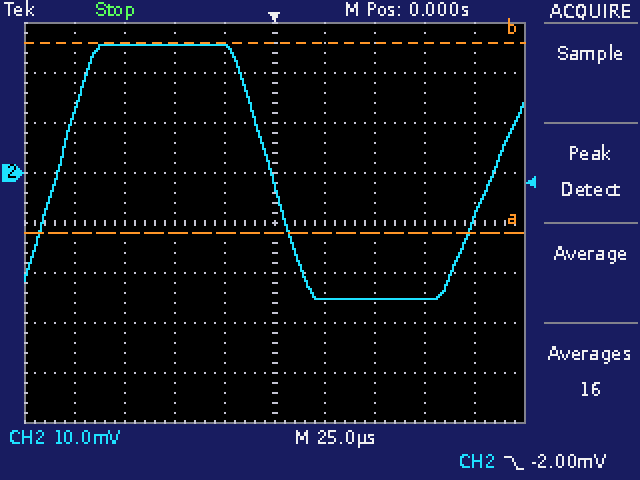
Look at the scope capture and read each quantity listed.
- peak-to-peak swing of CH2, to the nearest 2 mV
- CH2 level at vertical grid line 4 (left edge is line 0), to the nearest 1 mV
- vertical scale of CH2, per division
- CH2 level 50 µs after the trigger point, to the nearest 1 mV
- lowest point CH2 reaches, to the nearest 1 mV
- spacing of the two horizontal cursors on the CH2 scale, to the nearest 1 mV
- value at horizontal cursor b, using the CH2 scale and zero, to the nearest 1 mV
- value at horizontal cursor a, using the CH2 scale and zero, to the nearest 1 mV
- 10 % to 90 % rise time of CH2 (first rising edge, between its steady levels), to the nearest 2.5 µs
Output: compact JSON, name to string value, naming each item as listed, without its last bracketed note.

{"peak-to-peak swing of CH2, to the nearest 2 mV": "50 mV", "CH2 level at vertical grid line 4 (left edge is line 0), to the nearest 1 mV": "25 mV", "vertical scale of CH2, per division": "10 mV", "CH2 level 50 µs after the trigger point, to the nearest 1 mV": "-25 mV", "lowest point CH2 reaches, to the nearest 1 mV": "-25 mV", "spacing of the two horizontal cursors on the CH2 scale, to the nearest 1 mV": "38 mV", "value at horizontal cursor b, using the CH2 scale and zero, to the nearest 1 mV": "26 mV", "value at horizontal cursor a, using the CH2 scale and zero, to the nearest 1 mV": "-12 mV", "10 % to 90 % rise time of CH2 (first rising edge, between its steady levels), to the nearest 2.5 µs": "30.0 µs"}
